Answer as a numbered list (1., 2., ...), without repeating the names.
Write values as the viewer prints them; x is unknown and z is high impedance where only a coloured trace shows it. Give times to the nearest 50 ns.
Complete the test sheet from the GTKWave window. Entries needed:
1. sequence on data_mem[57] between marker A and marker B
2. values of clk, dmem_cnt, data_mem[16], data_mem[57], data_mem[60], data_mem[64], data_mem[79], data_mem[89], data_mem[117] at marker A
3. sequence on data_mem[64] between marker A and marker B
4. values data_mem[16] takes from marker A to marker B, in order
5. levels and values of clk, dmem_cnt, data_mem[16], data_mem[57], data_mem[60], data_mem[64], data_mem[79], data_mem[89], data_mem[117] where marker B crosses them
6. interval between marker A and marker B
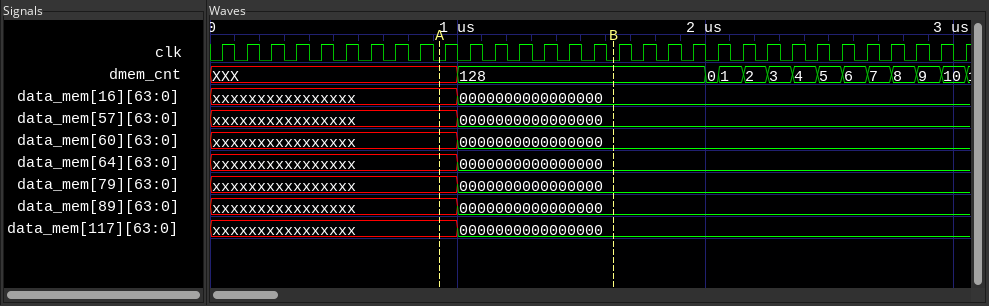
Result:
1. xxxxxxxxxxxxxxxx, 0000000000000000
2. clk=0, dmem_cnt=XXX, data_mem[16]=xxxxxxxxxxxxxxxx, data_mem[57]=xxxxxxxxxxxxxxxx, data_mem[60]=xxxxxxxxxxxxxxxx, data_mem[64]=xxxxxxxxxxxxxxxx, data_mem[79]=xxxxxxxxxxxxxxxx, data_mem[89]=xxxxxxxxxxxxxxxx, data_mem[117]=xxxxxxxxxxxxxxxx
3. xxxxxxxxxxxxxxxx, 0000000000000000
4. xxxxxxxxxxxxxxxx, 0000000000000000
5. clk=0, dmem_cnt=128, data_mem[16]=0000000000000000, data_mem[57]=0000000000000000, data_mem[60]=0000000000000000, data_mem[64]=0000000000000000, data_mem[79]=0000000000000000, data_mem[89]=0000000000000000, data_mem[117]=0000000000000000
6. 700 ns
